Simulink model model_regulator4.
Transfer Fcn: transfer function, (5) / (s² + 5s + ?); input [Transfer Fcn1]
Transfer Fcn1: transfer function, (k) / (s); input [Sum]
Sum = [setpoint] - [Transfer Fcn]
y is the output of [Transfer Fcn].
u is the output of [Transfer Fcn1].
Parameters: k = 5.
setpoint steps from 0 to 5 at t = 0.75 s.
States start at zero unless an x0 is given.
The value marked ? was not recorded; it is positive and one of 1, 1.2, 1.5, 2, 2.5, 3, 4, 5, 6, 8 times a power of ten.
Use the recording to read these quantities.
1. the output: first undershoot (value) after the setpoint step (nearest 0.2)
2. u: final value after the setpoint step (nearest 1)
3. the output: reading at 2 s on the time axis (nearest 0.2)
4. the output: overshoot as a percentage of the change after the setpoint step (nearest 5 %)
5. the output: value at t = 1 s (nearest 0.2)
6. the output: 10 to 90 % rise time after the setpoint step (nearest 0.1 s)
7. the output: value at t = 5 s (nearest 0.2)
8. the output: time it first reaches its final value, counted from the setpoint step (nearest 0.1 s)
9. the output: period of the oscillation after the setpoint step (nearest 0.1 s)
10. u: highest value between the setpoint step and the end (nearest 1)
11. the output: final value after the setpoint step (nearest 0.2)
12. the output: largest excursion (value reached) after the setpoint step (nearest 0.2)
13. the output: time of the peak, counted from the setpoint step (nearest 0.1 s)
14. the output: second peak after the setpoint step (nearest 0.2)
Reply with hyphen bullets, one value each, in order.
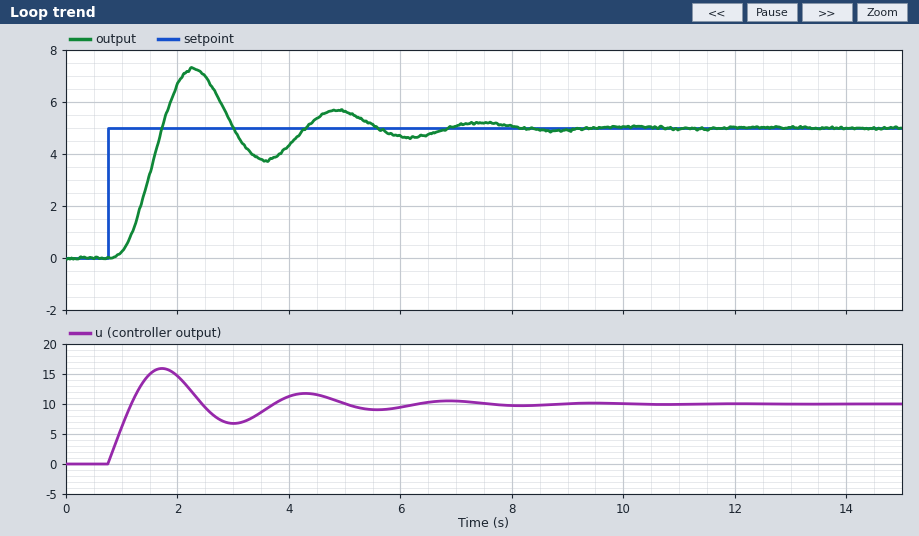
- 3.8
- 10
- 6.6
- 45 %
- 0.2
- 0.6 s
- 5.6
- 1.0 s
- 2.6 s
- 16
- 5.0
- 7.2
- 1.5 s
- 5.6
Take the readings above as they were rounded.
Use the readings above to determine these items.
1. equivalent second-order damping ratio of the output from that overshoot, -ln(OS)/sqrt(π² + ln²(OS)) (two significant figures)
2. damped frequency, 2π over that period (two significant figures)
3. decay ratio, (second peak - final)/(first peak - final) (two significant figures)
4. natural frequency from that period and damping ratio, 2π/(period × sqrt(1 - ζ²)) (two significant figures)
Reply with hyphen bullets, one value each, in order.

- 0.25
- 2.4 rad/s
- 0.27
- 2.5 rad/s
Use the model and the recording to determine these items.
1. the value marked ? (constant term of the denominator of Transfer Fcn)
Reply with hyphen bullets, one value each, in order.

- 10
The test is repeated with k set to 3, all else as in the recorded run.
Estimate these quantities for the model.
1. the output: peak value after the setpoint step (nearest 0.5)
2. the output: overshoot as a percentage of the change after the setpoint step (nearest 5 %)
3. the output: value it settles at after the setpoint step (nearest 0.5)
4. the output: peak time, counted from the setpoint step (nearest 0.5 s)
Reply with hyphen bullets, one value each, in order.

- 6.0
- 20 %
- 5.0
- 2.0 s
